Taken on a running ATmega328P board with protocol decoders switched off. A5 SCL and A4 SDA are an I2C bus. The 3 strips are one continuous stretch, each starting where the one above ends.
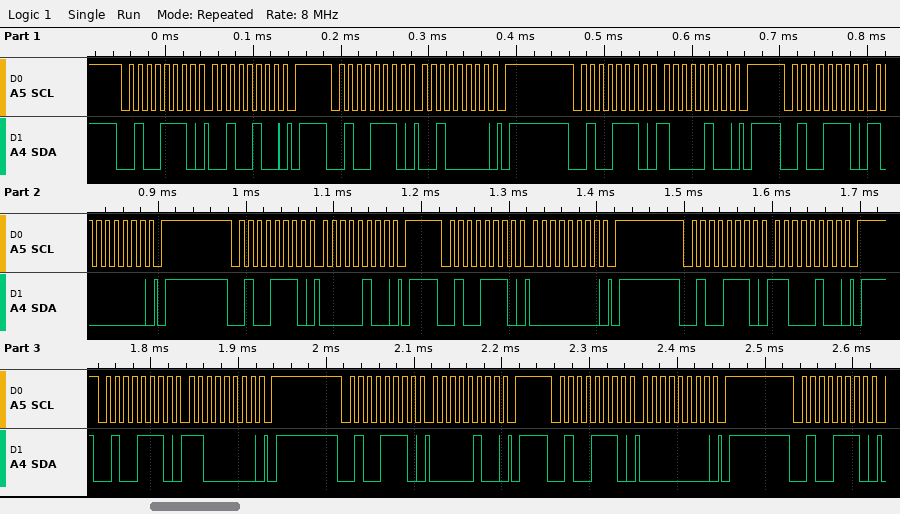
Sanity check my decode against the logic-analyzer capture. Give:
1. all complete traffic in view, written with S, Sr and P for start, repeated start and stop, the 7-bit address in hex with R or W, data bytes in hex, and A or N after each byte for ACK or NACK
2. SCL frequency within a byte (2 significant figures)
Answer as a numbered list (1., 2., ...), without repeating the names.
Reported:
1. S 27W A 24 A P S 27W A 20 A P S 27W A 84 A P S 27W A 80 A P S 27W A 04 A P S 27W A 00 A P S 27W A C4 A P S 27W A C0 A P S 27W A 04 A P S 27W A 00 A P S 27W A
2. 100 kHz
